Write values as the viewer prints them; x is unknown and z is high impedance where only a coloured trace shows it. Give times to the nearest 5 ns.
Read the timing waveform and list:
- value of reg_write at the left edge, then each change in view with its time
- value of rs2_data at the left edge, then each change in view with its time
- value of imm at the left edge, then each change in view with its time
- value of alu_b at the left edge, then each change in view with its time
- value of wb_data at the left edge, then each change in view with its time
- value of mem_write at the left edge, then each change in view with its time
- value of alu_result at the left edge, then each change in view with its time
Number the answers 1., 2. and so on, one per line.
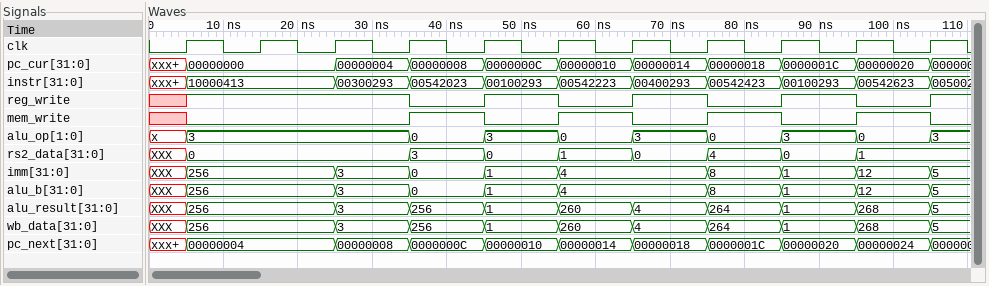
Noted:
1. x, 1 at 5 ns, 0 at 35 ns, 1 at 45 ns, 0 at 55 ns, 1 at 65 ns, 0 at 75 ns, 1 at 85 ns, 0 at 95 ns, 1 at 105 ns
2. XXX, 0 at 5 ns, 3 at 35 ns, 0 at 45 ns, 1 at 55 ns, 0 at 65 ns, 4 at 75 ns, 0 at 85 ns, 1 at 95 ns
3. XXX, 256 at 5 ns, 3 at 25 ns, 0 at 35 ns, 1 at 45 ns, 4 at 55 ns, 8 at 75 ns, 1 at 85 ns, 12 at 95 ns, 5 at 105 ns
4. XXX, 256 at 5 ns, 3 at 25 ns, 0 at 35 ns, 1 at 45 ns, 4 at 55 ns, 8 at 75 ns, 1 at 85 ns, 12 at 95 ns, 5 at 105 ns
5. XXX, 256 at 5 ns, 3 at 25 ns, 256 at 35 ns, 1 at 45 ns, 260 at 55 ns, 4 at 65 ns, 264 at 75 ns, 1 at 85 ns, 268 at 95 ns, 5 at 105 ns
6. x, 0 at 5 ns, 1 at 35 ns, 0 at 45 ns, 1 at 55 ns, 0 at 65 ns, 1 at 75 ns, 0 at 85 ns, 1 at 95 ns, 0 at 105 ns
7. XXX, 256 at 5 ns, 3 at 25 ns, 256 at 35 ns, 1 at 45 ns, 260 at 55 ns, 4 at 65 ns, 264 at 75 ns, 1 at 85 ns, 268 at 95 ns, 5 at 105 ns
